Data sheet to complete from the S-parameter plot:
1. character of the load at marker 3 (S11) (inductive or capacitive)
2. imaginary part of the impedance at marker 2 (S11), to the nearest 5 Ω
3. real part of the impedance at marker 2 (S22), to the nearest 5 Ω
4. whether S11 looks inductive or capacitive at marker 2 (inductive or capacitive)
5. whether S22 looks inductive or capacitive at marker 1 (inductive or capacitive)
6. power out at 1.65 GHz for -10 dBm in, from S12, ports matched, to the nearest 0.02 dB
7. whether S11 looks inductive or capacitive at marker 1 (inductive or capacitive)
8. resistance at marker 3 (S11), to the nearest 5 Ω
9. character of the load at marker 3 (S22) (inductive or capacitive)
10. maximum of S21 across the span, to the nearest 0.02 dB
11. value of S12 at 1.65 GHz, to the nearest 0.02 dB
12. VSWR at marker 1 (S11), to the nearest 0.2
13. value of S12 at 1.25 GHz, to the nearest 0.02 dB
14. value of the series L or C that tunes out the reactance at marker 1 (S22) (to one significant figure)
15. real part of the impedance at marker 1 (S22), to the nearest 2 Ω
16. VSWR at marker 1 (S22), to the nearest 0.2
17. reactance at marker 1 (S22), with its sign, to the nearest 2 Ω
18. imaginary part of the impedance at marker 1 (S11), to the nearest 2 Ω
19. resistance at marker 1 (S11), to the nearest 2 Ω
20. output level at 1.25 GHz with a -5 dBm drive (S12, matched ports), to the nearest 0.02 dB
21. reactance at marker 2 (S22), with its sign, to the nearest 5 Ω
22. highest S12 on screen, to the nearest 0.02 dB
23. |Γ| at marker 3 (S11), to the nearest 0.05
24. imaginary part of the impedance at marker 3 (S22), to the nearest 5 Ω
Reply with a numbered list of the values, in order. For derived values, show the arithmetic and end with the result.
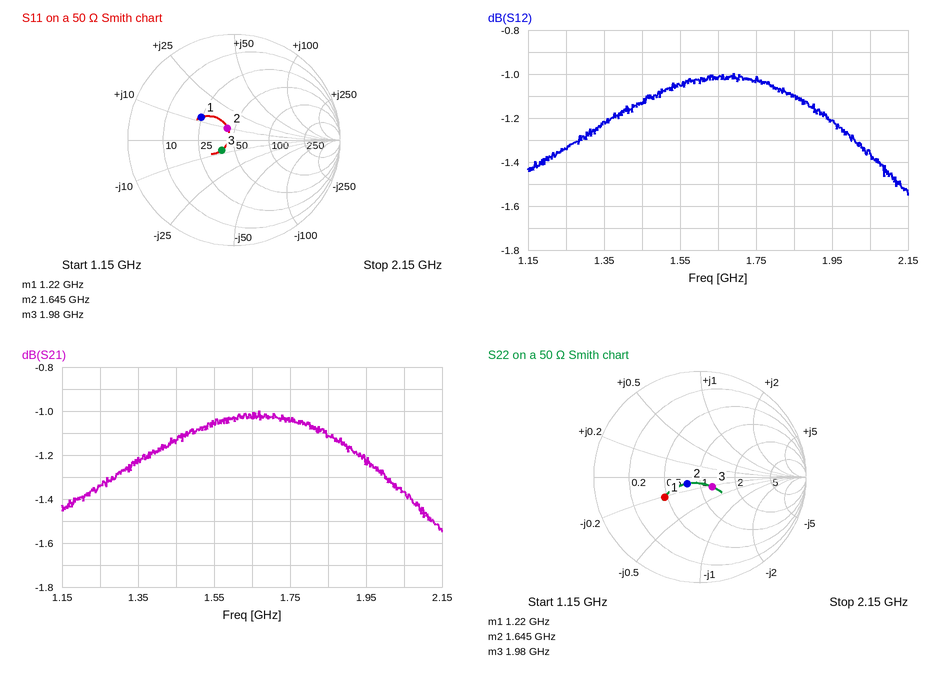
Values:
1. capacitive
2. +10 Ω
3. 40 Ω
4. inductive
5. capacitive
6. -10 dBm + (-1.02 dB) = -11.02 dBm
7. inductive
8. 40 Ω
9. capacitive
10. -1.00 dB
11. -1.02 dB
12. 2.2
13. -1.34 dB
14. L = 10 Ω/(2π × 1.22 GHz) ≈ 1 nH
15. 24 Ω
16. 2.2
17. -10 Ω
18. +12 Ω
19. 24 Ω
20. -5 dBm + (-1.34 dB) = -6.34 dBm
21. -5 Ω
22. -1.00 dB
23. 0.15
24. -10 Ω
